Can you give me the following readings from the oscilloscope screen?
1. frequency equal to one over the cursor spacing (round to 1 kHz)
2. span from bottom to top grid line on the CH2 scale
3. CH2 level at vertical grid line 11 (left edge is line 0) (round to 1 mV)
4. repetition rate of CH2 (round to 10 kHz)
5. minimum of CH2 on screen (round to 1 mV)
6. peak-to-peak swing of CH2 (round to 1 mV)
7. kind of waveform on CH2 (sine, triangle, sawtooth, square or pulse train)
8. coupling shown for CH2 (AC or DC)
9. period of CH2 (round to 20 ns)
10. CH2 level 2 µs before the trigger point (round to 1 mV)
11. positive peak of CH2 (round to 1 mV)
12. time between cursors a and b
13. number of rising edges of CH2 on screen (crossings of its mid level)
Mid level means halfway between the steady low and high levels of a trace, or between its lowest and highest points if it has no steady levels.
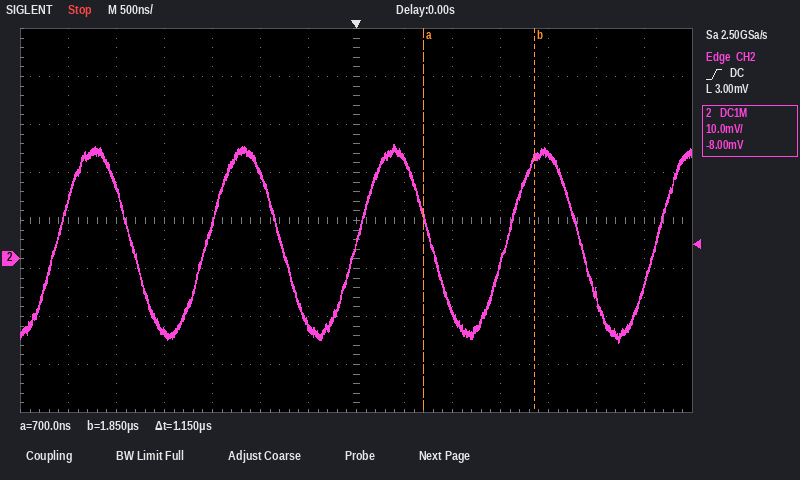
870 kHz
80 mV
22 mV
640 kHz
-17 mV
41 mV
sine
DC
1.56 µs
-15 mV
24 mV
1.15 µs
5
